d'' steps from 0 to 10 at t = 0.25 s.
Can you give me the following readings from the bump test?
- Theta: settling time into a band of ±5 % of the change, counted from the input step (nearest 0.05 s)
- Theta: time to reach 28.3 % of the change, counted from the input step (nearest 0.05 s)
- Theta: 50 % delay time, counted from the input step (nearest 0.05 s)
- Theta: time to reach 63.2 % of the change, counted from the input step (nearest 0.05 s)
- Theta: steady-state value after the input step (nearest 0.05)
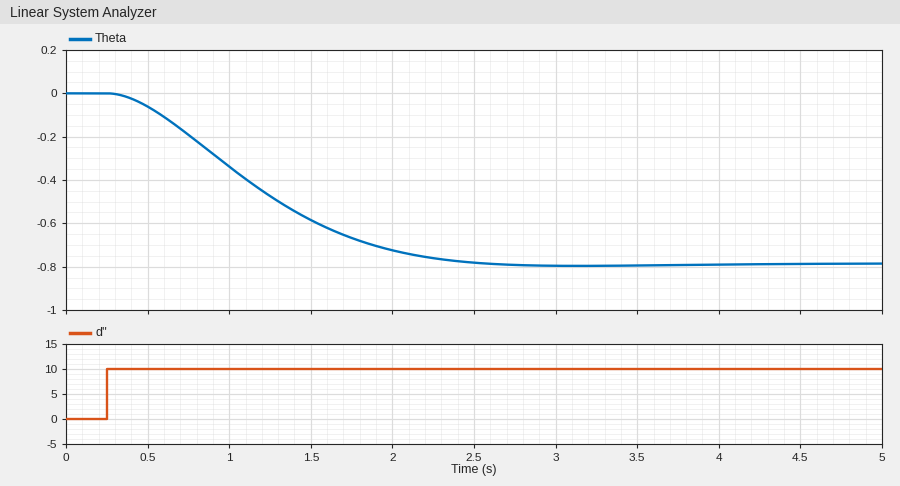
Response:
1.90 s
0.55 s
0.85 s
1.05 s
-0.80
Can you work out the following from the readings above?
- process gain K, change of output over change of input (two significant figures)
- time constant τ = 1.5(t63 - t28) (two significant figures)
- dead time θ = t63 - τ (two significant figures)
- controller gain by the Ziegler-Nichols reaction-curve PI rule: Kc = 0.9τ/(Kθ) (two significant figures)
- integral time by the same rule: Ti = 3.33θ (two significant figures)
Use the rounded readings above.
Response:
-0.080
0.75 s
0.30 s
-28
1.00 s
